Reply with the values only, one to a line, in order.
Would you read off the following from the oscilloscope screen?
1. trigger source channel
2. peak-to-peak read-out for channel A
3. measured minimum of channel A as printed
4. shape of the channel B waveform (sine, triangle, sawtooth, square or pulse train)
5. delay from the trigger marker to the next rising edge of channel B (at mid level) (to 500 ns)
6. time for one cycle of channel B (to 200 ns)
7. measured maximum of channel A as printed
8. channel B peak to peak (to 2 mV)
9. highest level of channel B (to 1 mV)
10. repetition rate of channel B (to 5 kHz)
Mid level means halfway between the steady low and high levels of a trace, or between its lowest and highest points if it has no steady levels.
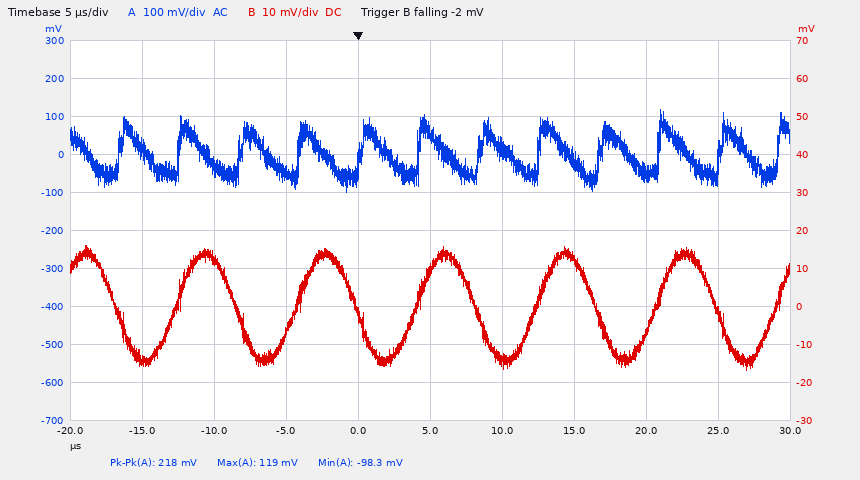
channel B
218 mV
-98.3 mV
sine
4.0 µs
8.4 µs
119 mV
32 mV
16 mV
120 kHz
